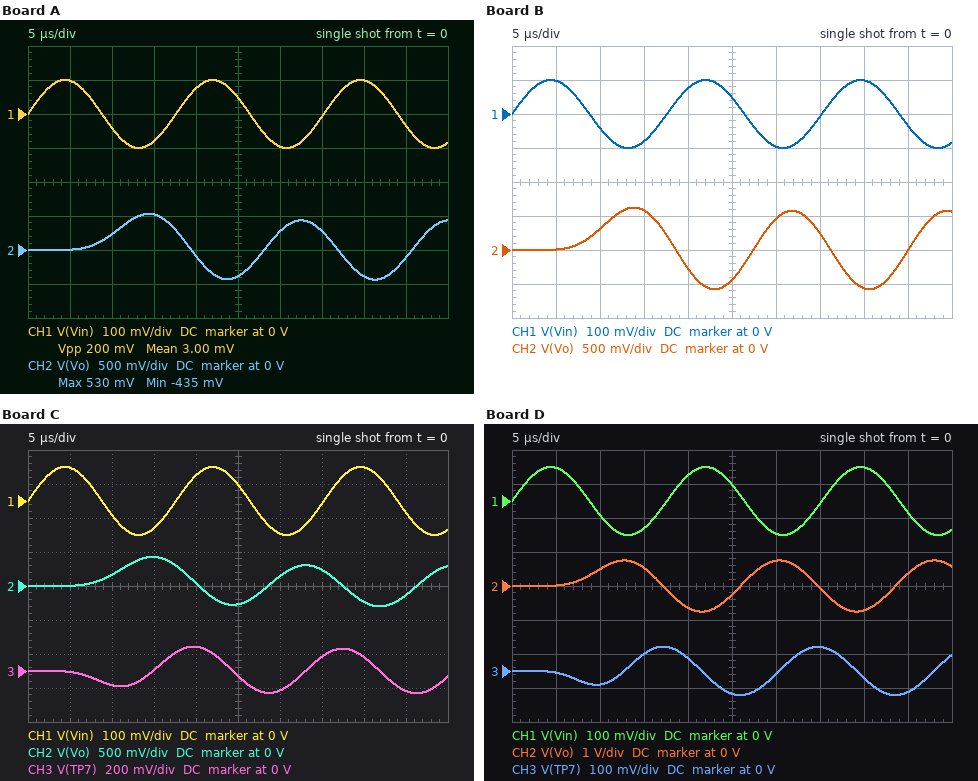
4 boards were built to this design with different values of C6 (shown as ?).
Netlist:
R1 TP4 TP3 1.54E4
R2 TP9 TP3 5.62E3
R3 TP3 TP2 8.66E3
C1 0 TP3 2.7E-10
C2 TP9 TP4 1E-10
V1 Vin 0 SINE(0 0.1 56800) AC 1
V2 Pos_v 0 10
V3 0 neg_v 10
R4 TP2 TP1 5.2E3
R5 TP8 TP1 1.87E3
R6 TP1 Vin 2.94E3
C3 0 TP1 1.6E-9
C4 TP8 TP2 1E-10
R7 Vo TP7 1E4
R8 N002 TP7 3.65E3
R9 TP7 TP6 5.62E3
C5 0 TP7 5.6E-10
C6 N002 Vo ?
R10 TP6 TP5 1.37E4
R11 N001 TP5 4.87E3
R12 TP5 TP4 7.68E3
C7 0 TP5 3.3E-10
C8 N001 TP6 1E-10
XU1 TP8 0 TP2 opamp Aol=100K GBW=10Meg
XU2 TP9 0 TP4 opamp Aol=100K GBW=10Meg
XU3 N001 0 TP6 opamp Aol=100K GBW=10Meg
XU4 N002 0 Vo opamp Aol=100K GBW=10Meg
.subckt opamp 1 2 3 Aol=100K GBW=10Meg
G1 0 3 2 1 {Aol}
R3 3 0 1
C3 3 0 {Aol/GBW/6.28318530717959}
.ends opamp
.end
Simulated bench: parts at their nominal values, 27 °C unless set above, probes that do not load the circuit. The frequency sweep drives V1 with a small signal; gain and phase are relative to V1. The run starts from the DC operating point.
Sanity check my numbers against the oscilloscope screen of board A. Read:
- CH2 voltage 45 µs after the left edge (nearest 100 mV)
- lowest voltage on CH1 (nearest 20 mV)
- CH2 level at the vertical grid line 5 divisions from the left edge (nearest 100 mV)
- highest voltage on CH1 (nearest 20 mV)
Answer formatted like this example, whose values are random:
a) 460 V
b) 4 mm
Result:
a) -100 mV
b) -100 mV
c) -400 mV
d) 100 mV
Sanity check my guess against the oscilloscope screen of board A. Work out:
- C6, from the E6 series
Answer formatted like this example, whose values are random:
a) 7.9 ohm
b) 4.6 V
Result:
a) 220 pF
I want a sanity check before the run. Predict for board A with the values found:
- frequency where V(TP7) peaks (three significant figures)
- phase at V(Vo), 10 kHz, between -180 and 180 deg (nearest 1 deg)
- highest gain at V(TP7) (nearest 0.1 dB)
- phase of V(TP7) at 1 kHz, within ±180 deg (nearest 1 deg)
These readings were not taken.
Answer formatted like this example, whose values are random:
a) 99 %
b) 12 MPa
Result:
a) 46.0 kHz
b) -41 deg
c) 2.4 dB
d) -94 deg
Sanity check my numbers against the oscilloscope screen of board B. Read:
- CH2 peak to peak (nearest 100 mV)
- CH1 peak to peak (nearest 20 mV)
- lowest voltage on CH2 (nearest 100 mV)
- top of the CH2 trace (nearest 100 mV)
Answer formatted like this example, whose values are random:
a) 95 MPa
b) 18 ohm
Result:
a) 1.2 V
b) 200 mV
c) -600 mV
d) 600 mV
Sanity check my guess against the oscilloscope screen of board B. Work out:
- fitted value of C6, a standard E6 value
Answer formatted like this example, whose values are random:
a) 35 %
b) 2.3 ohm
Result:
a) 150 pF
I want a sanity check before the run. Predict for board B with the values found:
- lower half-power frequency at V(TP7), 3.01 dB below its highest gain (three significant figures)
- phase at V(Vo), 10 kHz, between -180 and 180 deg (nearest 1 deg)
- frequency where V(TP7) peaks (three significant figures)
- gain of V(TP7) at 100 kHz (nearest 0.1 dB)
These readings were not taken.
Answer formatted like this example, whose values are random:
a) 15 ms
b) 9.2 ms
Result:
a) 26.2 kHz
b) -36 deg
c) 55.1 kHz
d) -2.9 dB
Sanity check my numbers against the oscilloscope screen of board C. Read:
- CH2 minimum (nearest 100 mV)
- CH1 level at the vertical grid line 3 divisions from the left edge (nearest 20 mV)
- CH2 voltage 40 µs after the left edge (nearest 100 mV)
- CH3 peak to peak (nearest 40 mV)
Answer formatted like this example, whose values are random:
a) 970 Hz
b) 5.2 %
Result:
a) -300 mV
b) -80 mV
c) -200 mV
d) 280 mV
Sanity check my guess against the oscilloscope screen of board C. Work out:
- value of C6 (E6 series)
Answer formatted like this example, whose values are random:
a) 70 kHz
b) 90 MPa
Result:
a) 330 pF
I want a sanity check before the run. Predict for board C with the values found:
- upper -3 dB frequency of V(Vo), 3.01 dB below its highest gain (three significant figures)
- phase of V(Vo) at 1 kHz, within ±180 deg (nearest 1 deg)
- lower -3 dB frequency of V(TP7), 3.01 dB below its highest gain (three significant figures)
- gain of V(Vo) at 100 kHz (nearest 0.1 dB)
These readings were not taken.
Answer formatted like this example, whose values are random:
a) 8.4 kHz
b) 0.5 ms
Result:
a) 24.4 kHz
b) -5 deg
c) 15.9 kHz
d) -1.3 dB
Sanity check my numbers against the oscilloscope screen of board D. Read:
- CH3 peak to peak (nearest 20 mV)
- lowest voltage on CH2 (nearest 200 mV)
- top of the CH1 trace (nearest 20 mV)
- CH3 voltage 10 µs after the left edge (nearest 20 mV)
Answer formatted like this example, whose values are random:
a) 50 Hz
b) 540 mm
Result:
a) 140 mV
b) -800 mV
c) 100 mV
d) -40 mV
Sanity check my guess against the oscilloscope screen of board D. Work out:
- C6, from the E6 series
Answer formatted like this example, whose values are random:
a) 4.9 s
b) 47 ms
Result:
a) 68 pF
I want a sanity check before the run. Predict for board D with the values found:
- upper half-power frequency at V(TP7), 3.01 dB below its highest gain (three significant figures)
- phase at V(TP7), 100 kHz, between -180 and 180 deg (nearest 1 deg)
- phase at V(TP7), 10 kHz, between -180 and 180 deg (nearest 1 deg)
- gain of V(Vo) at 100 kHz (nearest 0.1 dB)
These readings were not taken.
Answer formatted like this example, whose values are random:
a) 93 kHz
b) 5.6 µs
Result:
a) 113 kHz
b) -35 deg
c) -120 deg
d) 12.1 dB
